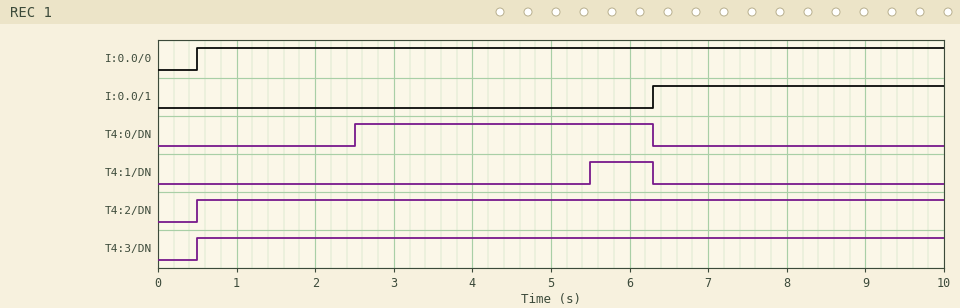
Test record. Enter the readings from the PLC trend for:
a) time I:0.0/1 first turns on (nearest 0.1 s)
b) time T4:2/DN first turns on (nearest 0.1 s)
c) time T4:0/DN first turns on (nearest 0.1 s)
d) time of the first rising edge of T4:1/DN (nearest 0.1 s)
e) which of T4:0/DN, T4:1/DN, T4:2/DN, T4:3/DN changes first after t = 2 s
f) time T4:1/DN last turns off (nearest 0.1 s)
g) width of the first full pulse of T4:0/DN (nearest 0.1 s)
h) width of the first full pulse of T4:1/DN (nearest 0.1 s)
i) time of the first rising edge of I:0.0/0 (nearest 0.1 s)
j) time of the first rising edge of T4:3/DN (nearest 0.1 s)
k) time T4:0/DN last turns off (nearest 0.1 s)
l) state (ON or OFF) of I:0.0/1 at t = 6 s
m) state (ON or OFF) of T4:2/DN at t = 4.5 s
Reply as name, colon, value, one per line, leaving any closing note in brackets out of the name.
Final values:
time I:0.0/1 first turns on: 6.3 s
time T4:2/DN first turns on: 0.5 s
time T4:0/DN first turns on: 2.5 s
time of the first rising edge of T4:1/DN: 5.5 s
which of T4:0/DN, T4:1/DN, T4:2/DN, T4:3/DN changes first after t = 2 s: T4:0/DN
time T4:1/DN last turns off: 6.3 s
width of the first full pulse of T4:0/DN: 3.8 s
width of the first full pulse of T4:1/DN: 0.8 s
time of the first rising edge of I:0.0/0: 0.5 s
time of the first rising edge of T4:3/DN: 0.5 s
time T4:0/DN last turns off: 6.3 s
state (ON or OFF) of I:0.0/1 at t = 6 s: OFF
state (ON or OFF) of T4:2/DN at t = 4.5 s: ON
